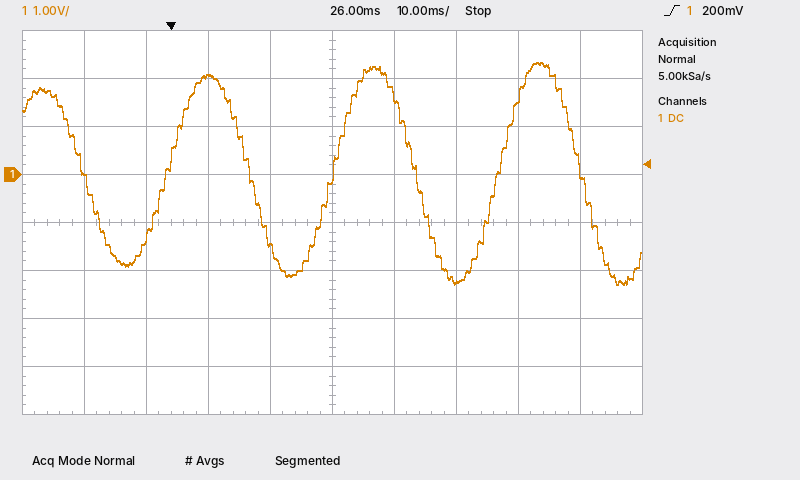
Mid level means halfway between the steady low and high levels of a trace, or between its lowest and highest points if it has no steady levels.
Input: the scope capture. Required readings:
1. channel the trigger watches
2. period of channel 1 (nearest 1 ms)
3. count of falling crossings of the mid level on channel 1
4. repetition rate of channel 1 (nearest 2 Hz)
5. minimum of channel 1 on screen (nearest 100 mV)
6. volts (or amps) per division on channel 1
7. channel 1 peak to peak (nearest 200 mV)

channel 1
27 ms
4
38 Hz
-2.3 V
1 V
4.6 V
